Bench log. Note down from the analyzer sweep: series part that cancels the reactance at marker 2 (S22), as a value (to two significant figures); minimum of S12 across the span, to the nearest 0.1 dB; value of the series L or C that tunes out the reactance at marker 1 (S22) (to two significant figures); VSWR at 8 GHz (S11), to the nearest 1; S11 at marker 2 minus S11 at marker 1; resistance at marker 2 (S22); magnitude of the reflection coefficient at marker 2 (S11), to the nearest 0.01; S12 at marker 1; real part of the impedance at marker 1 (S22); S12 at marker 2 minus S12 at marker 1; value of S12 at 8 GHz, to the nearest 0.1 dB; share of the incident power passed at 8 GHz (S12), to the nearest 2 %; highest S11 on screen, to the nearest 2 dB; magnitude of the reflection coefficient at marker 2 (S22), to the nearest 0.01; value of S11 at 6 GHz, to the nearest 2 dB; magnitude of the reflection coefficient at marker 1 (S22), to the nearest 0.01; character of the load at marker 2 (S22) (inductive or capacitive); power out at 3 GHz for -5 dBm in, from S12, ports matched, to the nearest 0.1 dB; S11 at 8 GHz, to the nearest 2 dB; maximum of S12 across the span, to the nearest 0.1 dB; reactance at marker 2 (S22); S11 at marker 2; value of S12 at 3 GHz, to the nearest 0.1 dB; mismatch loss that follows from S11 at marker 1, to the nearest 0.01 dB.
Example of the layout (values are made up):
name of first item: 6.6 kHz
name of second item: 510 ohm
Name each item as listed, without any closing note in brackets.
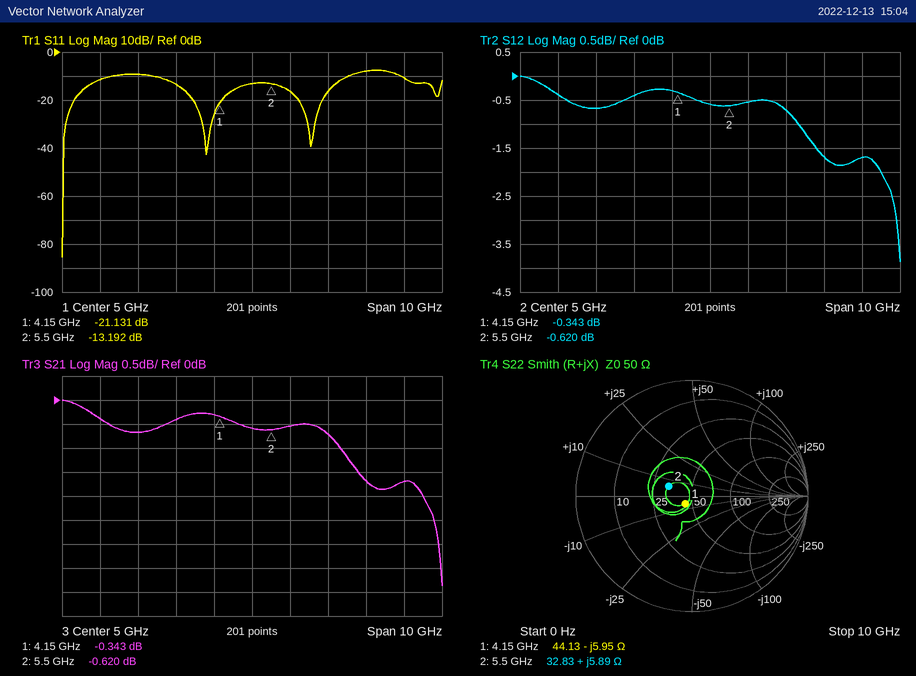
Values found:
series part that cancels the reactance at marker 2 (S22), as a value: 4.9 pF
minimum of S12 across the span, to the nearest 0.1 dB: -3.9 dB
value of the series L or C that tunes out the reactance at marker 1 (S22): 230 pH
VSWR at 8 GHz (S11), to the nearest 1: 2
S11 at marker 2 minus S11 at marker 1: 7.939 dB
resistance at marker 2: 32.83 Ω
magnitude of the reflection coefficient at marker 2 (S11), to the nearest 0.01: 0.22
S12 at marker 1: -0.343 dB
real part of the impedance at marker 1: 44.13 Ω
S12 at marker 2 minus S12 at marker 1: -0.277 dB
value of S12 at 8 GHz, to the nearest 0.1 dB: -1.7 dB
share of the incident power passed at 8 GHz (S12), to the nearest 2 %: 68 %
highest S11 on screen, to the nearest 2 dB: -8 dB
magnitude of the reflection coefficient at marker 2 (S22), to the nearest 0.01: 0.22
value of S11 at 6 GHz, to the nearest 2 dB: -16 dB
magnitude of the reflection coefficient at marker 1 (S22), to the nearest 0.01: 0.09
character of the load at marker 2 (S22): inductive
power out at 3 GHz for -5 dBm in, from S12, ports matched, to the nearest 0.1 dB: -5.4 dBm
S11 at 8 GHz, to the nearest 2 dB: -8 dB
maximum of S12 across the span, to the nearest 0.1 dB: 0.0 dB
reactance at marker 2: +5.89 Ω
S11 at marker 2: -13.192 dB
value of S12 at 3 GHz, to the nearest 0.1 dB: -0.4 dB
mismatch loss that follows from S11 at marker 1, to the nearest 0.01 dB: 0.03 dB
